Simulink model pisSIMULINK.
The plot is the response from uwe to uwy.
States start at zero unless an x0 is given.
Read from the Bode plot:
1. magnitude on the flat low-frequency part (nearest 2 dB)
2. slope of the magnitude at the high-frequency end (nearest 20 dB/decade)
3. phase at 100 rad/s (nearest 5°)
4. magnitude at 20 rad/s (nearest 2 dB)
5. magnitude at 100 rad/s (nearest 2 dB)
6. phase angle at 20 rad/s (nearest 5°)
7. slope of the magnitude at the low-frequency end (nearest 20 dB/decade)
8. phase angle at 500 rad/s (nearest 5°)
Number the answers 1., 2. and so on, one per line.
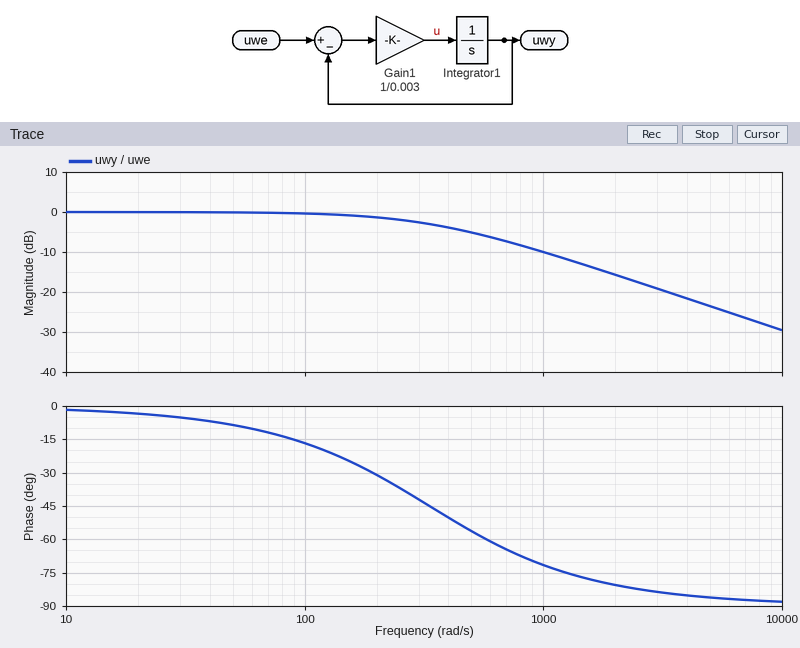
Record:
1. 0 dB
2. -20 dB/decade
3. -15°
4. 0 dB
5. 0 dB
6. -5°
7. 0 dB/decade
8. -55°
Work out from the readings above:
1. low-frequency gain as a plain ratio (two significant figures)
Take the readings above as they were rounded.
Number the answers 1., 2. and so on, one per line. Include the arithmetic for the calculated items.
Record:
1. 10^(0 / 20) = 1.0
